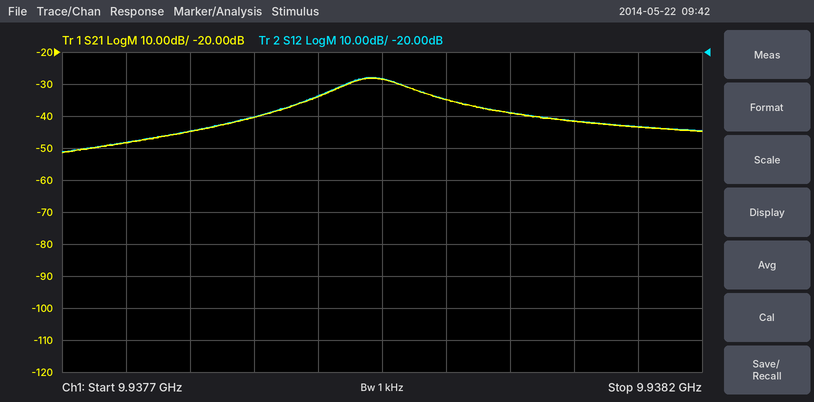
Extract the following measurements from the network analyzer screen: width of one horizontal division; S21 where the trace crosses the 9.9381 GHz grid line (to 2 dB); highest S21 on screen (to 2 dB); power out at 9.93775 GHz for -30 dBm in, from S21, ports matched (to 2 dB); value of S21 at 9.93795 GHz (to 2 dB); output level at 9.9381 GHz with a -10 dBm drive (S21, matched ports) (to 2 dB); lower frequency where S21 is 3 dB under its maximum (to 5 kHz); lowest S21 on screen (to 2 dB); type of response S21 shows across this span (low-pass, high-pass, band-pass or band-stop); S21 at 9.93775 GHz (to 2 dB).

50 kHz
-42 dB
-28 dB
-78 dBm
-28 dB
-52 dBm
9.937915 GHz
-52 dB
band-pass
-48 dB
